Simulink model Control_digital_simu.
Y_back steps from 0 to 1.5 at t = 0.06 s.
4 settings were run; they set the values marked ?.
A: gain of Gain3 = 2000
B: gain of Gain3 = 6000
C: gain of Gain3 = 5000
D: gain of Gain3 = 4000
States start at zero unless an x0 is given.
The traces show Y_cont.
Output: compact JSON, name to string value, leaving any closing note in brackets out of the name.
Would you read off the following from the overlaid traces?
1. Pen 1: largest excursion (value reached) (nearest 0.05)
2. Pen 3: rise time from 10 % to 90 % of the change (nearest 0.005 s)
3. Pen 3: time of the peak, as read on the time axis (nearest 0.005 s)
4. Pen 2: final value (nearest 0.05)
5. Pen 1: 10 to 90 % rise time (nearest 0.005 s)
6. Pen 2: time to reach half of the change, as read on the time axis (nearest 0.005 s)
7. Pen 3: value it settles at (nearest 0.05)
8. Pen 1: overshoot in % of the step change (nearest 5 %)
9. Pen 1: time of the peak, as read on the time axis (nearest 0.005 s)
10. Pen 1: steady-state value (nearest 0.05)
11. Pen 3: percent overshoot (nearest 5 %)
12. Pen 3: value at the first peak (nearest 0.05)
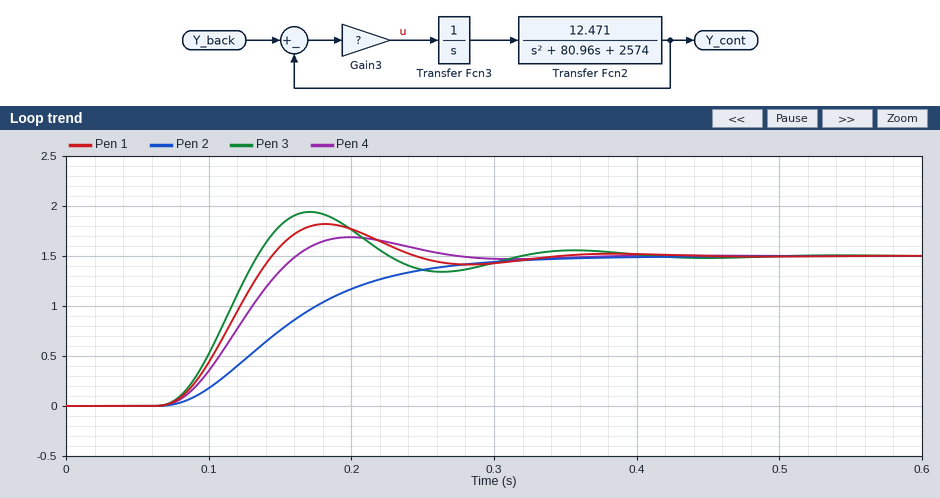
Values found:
{"Pen 1: largest excursion (value reached)": "1.80", "Pen 3: rise time from 10 % to 90 % of the change": "0.045 s", "Pen 3: time of the peak, as read on the time axis": "0.170 s", "Pen 2: final value": "1.50", "Pen 1: 10 to 90 % rise time": "0.050 s", "Pen 2: time to reach half of the change, as read on the time axis": "0.150 s", "Pen 3: value it settles at": "1.50", "Pen 1: overshoot in % of the step change": "20 %", "Pen 1: time of the peak, as read on the time axis": "0.180 s", "Pen 1: steady-state value": "1.50", "Pen 3: percent overshoot": "30 %", "Pen 3: value at the first peak": "1.95"}
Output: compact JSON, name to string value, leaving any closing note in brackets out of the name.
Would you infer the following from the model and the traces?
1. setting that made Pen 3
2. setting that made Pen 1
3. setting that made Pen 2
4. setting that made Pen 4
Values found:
{"setting that made Pen 3": "B", "setting that made Pen 1": "C", "setting that made Pen 2": "A", "setting that made Pen 4": "D"}
